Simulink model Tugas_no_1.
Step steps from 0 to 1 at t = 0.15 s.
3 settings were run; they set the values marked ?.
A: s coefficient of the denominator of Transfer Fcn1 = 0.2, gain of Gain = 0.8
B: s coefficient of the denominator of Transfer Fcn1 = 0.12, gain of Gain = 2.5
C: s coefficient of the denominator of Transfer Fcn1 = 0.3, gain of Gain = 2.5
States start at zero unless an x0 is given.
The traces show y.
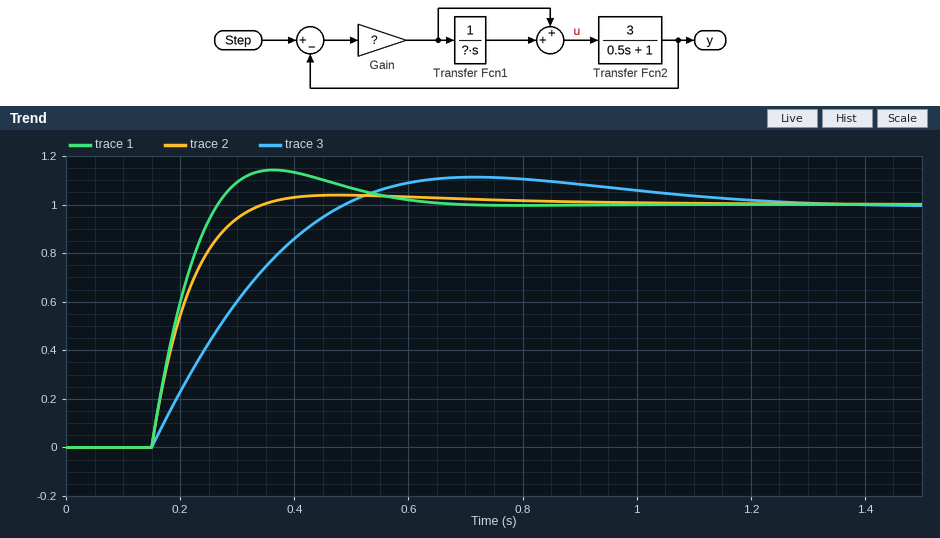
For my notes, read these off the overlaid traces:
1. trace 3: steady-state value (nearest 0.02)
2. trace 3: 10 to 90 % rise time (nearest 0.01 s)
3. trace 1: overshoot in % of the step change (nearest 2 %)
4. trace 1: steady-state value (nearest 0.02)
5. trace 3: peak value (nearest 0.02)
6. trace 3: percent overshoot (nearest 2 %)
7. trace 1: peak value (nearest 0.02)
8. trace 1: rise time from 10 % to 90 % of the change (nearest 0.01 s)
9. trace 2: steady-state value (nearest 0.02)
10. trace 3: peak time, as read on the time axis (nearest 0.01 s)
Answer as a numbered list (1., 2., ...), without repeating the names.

1. 1.00
2. 0.25 s
3. 14 %
4. 1.00
5. 1.12
6. 12 %
7. 1.14
8. 0.09 s
9. 1.00
10. 0.72 s
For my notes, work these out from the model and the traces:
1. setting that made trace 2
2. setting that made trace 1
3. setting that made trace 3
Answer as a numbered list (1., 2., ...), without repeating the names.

1. C
2. B
3. A
